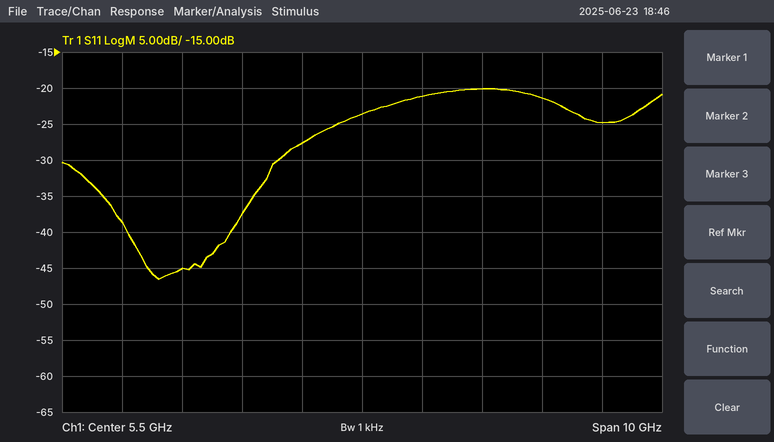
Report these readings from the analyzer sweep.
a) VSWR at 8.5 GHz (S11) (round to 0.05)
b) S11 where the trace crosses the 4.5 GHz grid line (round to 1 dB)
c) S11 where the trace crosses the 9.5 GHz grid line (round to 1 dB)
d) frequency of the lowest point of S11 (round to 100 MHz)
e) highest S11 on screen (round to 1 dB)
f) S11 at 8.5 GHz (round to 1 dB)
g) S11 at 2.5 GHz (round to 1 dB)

1.20
-28 dB
-25 dB
2.1 GHz
-20 dB
-21 dB
-45 dB
